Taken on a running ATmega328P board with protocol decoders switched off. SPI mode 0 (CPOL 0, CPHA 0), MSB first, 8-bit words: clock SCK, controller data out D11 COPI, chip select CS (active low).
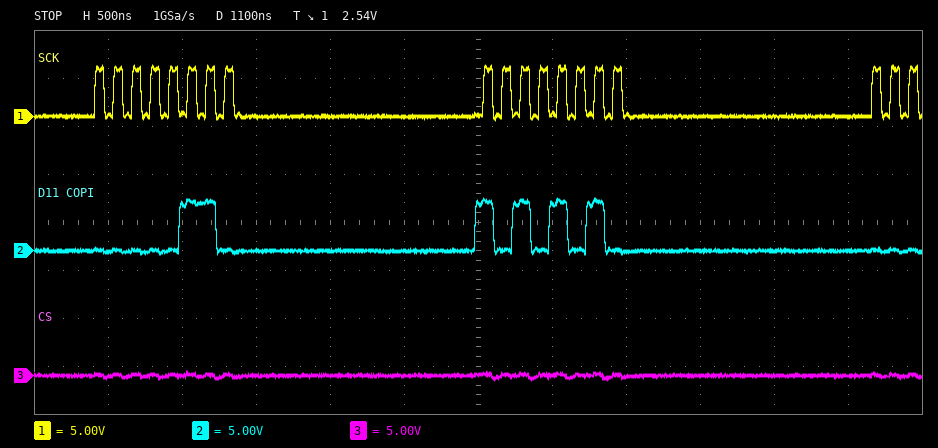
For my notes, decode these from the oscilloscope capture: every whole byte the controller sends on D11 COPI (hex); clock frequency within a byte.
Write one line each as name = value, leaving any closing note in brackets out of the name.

every whole byte the controller sends on D11 COPI = 06 AA
clock frequency within a byte = 8 MHz
